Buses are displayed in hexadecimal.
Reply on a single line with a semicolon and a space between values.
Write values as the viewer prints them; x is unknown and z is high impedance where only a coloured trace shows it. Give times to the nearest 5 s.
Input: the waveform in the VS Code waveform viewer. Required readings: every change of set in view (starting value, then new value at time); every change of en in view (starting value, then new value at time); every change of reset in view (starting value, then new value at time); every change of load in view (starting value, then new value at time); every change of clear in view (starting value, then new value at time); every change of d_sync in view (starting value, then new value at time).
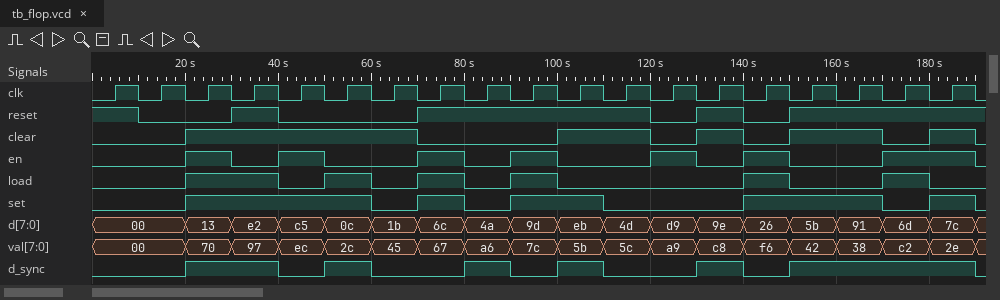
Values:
0, 1 at 20 s, 0 at 60 s, 1 at 70 s, 0 at 80 s, 1 at 90 s, 0 at 110 s, 1 at 140 s, 0 at 170 s, 1 at 180 s, 0 at 190 s; 0, 1 at 20 s, 0 at 30 s, 1 at 40 s, 0 at 50 s, 1 at 70 s, 0 at 80 s, 1 at 90 s, 0 at 100 s, 1 at 120 s, 0 at 130 s, 1 at 140 s, 0 at 150 s, 1 at 170 s, 0 at 190 s; 1, 0 at 10 s, 1 at 30 s, 0 at 40 s, 1 at 70 s, 0 at 120 s, 1 at 130 s, 0 at 140 s, 1 at 150 s; 0, 1 at 20 s, 0 at 40 s, 1 at 50 s, 0 at 60 s, 1 at 70 s, 0 at 80 s, 1 at 90 s, 0 at 100 s, 1 at 140 s, 0 at 150 s, 1 at 170 s, 0 at 180 s; 0, 1 at 20 s, 0 at 70 s, 1 at 100 s, 0 at 120 s, 1 at 130 s, 0 at 140 s, 1 at 150 s, 0 at 170 s, 1 at 180 s, 0 at 190 s; 0, 1 at 20 s, 0 at 40 s, 1 at 50 s, 0 at 60 s, 1 at 80 s, 0 at 90 s, 1 at 100 s, 0 at 110 s, 1 at 130 s, 0 at 140 s, 1 at 150 s, 0 at 190 s
